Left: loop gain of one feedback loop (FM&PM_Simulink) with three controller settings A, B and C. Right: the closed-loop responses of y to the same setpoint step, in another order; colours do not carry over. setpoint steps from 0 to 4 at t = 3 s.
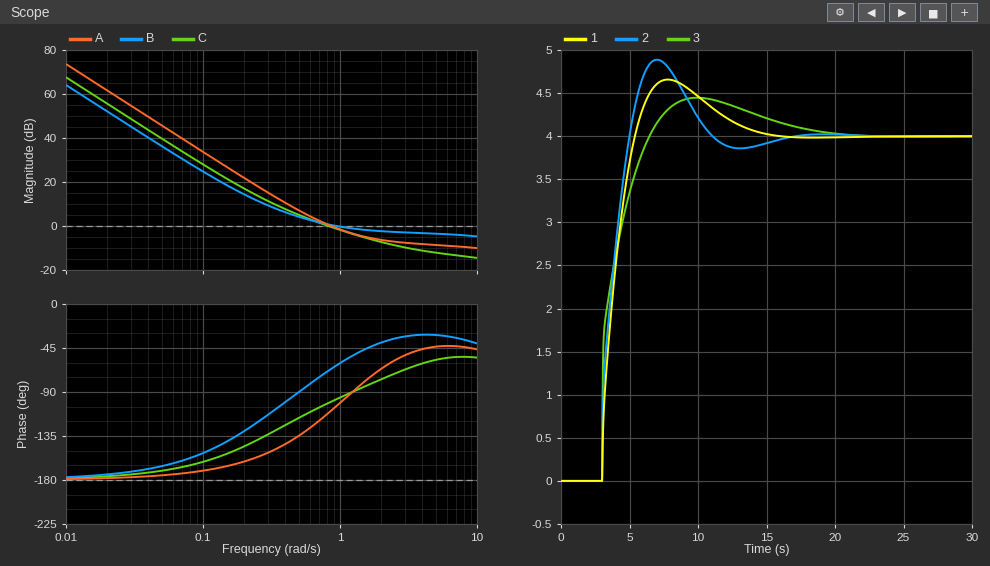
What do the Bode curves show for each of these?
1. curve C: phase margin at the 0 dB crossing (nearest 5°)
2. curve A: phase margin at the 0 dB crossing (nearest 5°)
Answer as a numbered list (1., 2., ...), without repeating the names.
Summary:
1. 80°
2. 70°
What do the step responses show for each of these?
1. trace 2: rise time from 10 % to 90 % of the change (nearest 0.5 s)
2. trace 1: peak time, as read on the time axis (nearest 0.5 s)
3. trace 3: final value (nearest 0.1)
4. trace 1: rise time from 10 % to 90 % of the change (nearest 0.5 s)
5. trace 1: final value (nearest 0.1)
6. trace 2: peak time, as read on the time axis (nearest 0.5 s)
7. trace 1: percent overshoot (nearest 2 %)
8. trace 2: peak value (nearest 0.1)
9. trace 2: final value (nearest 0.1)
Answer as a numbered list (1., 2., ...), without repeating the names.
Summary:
1. 1.5 s
2. 8.0 s
3. 4.0
4. 2.0 s
5. 4.0
6. 7.0 s
7. 16 %
8. 4.9
9. 4.0
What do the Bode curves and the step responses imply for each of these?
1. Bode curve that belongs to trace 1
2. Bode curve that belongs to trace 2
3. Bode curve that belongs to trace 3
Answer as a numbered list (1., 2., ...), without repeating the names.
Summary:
1. C
2. A
3. B
